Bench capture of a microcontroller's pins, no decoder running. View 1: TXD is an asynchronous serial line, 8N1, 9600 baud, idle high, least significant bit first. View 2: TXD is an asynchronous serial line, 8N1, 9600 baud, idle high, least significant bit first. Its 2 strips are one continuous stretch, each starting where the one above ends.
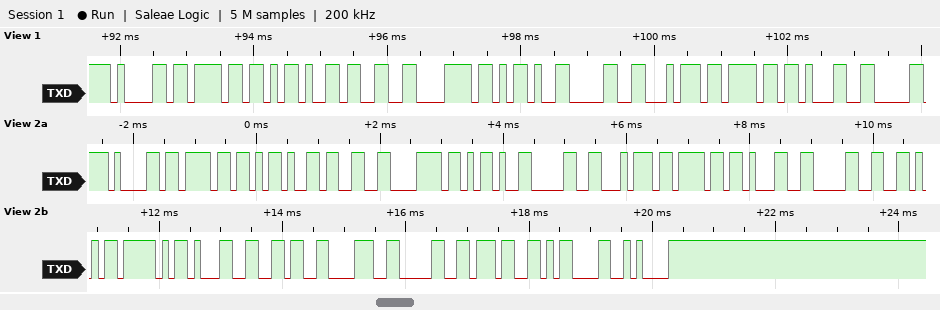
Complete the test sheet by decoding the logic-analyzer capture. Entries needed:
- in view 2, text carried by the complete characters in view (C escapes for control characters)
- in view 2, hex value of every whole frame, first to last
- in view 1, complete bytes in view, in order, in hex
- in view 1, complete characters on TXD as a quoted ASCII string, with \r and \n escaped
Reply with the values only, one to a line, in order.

"ao-3x-0to10V_16807\r\n"
61 6F 2D 33 78 2D 30 74 6F 31 30 56 5F 31 36 38 30 37 0D 0A
0x61 0x6F 0x2D 0x33 0x78 0x2D 0x30 0x74 0x6F 0x31
"ao-3x-0to1"
